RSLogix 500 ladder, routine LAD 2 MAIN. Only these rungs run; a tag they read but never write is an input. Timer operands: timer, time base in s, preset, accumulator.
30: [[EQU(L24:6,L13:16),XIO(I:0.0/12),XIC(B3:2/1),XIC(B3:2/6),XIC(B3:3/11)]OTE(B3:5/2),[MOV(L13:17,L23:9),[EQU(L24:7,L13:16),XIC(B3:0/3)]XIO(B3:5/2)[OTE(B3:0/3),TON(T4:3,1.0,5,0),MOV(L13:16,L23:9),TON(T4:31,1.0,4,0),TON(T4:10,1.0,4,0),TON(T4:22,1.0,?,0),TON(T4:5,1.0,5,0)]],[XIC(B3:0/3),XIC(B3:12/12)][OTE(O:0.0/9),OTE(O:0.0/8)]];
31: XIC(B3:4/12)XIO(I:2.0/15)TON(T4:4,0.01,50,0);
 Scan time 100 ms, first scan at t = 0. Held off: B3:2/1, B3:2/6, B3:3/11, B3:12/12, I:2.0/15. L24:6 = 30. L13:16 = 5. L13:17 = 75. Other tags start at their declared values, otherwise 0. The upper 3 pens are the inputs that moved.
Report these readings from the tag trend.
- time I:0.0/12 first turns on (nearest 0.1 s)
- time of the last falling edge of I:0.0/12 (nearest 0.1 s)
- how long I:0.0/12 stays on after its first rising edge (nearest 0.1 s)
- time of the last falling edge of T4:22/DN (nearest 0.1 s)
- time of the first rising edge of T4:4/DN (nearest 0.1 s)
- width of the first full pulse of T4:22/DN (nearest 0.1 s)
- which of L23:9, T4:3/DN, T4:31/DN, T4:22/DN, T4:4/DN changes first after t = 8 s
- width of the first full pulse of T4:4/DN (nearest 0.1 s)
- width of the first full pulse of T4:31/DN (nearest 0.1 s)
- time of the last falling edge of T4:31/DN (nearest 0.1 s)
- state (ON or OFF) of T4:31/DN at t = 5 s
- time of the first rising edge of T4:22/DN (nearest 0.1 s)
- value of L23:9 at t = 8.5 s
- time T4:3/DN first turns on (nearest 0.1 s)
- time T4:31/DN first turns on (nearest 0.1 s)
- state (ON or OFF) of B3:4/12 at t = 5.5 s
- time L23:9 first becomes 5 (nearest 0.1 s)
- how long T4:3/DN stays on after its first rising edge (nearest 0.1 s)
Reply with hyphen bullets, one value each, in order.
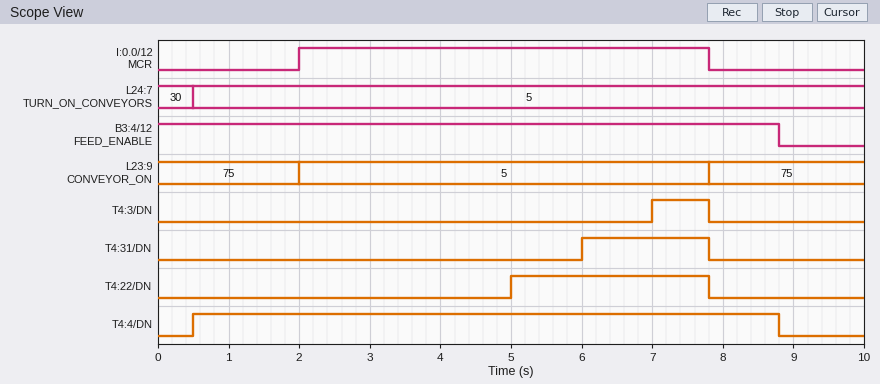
- 2.0 s
- 7.8 s
- 5.8 s
- 7.8 s
- 0.5 s
- 2.8 s
- T4:4/DN
- 8.3 s
- 1.8 s
- 7.8 s
- OFF
- 5.0 s
- 75
- 7.0 s
- 6.0 s
- ON
- 2.0 s
- 0.8 s
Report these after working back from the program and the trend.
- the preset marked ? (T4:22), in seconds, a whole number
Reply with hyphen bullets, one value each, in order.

- 3 s
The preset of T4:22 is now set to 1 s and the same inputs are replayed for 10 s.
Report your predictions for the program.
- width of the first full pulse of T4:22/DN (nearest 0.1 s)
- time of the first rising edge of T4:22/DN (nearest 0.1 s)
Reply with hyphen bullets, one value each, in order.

- 4.8 s
- 3.0 s
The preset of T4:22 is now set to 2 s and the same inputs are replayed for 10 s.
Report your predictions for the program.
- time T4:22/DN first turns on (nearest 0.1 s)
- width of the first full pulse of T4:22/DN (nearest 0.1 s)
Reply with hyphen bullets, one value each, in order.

- 4.0 s
- 3.8 s
